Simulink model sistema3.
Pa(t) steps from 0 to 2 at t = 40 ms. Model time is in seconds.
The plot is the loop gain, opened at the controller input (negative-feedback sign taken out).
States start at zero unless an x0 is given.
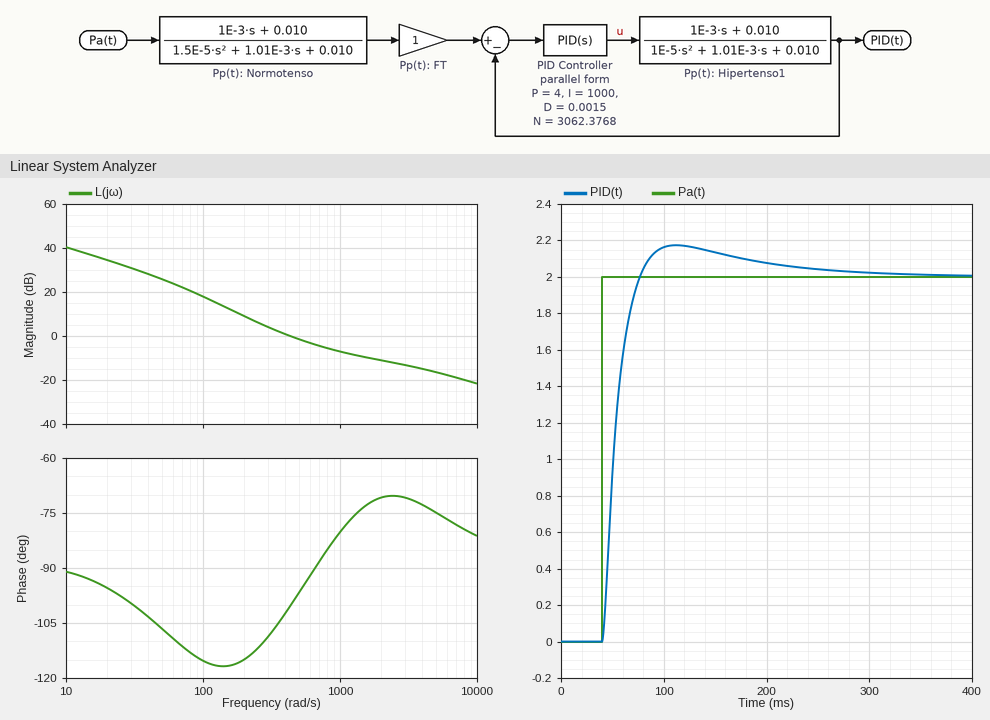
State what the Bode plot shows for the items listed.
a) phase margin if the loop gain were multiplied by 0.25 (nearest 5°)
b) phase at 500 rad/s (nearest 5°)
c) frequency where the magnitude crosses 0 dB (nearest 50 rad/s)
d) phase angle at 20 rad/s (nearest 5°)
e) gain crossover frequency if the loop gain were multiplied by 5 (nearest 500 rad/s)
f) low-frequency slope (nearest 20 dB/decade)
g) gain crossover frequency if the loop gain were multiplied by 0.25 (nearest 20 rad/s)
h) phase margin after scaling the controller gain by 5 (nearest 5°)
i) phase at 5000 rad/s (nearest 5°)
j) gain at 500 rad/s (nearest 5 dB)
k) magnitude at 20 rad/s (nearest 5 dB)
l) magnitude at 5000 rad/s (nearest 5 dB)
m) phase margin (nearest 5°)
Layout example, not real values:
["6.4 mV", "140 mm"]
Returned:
["65°", "-95°", "450 rad/s", "-95°", "3500 rad/s", "-20 dB/decade", "160 rad/s", "110°", "-75°", "0 dB", "35 dB", "-15 dB", "80°"]
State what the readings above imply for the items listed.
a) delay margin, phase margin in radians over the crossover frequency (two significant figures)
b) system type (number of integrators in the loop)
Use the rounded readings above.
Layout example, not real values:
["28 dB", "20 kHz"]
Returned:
["0.0031 s", "1"]
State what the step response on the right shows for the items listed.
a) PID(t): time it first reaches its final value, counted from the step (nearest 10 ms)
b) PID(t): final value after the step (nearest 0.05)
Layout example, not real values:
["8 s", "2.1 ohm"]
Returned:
["40 ms", "2.00"]
